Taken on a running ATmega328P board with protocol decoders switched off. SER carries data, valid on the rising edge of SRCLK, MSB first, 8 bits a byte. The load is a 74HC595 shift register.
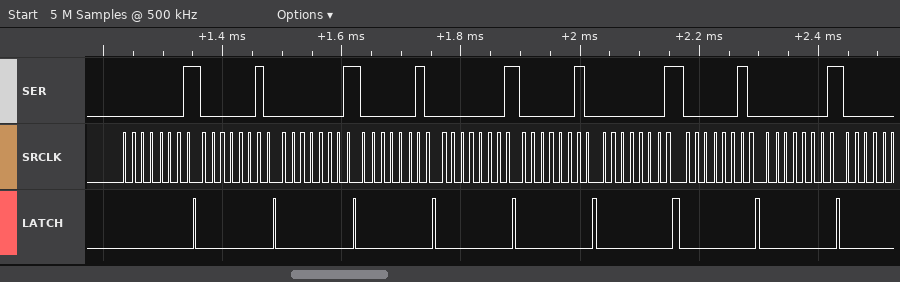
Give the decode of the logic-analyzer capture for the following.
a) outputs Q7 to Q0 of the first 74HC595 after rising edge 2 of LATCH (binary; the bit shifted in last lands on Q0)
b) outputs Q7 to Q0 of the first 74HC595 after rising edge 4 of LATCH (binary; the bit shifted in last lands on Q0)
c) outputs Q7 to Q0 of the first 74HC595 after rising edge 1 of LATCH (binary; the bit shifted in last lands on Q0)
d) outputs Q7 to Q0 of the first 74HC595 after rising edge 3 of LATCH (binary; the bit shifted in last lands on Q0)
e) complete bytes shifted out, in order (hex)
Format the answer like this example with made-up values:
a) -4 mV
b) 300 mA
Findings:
a) 00000010
b) 00000010
c) 00000001
d) 00000001
e) 01 02 01 02 01 02 01 02 01
